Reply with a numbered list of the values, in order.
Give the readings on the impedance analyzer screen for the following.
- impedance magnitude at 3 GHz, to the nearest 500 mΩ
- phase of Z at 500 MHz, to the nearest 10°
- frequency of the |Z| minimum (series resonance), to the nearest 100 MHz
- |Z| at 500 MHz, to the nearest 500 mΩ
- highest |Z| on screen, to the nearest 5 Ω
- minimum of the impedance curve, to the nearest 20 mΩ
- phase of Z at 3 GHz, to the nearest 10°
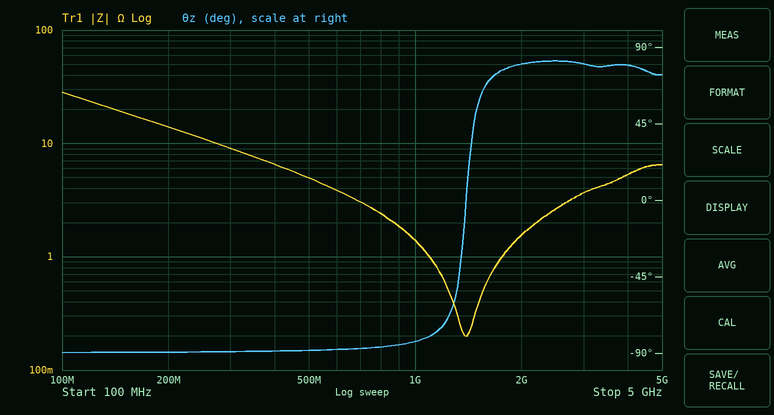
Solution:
1. 3.5 Ω
2. -90°
3. 1.4 GHz
4. 5.0 Ω
5. 30 Ω
6. 200 mΩ
7. 80°
